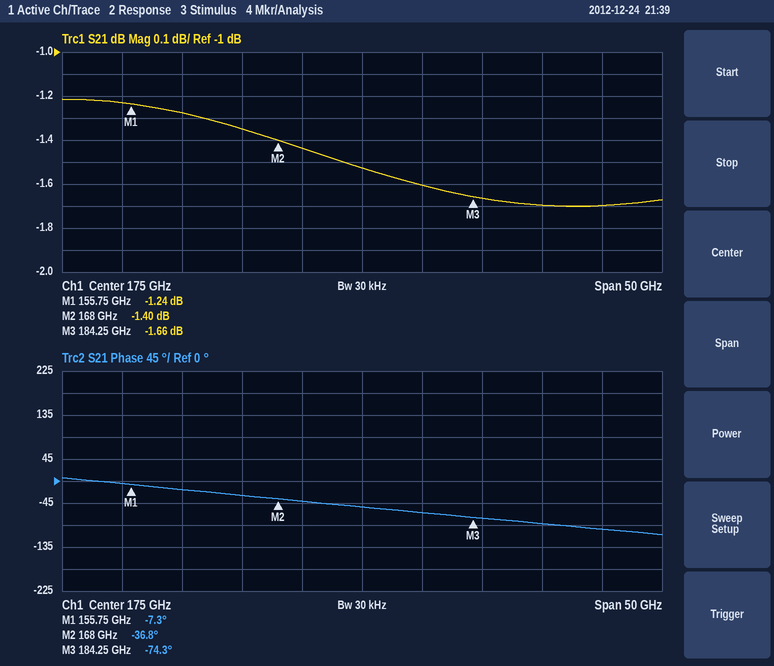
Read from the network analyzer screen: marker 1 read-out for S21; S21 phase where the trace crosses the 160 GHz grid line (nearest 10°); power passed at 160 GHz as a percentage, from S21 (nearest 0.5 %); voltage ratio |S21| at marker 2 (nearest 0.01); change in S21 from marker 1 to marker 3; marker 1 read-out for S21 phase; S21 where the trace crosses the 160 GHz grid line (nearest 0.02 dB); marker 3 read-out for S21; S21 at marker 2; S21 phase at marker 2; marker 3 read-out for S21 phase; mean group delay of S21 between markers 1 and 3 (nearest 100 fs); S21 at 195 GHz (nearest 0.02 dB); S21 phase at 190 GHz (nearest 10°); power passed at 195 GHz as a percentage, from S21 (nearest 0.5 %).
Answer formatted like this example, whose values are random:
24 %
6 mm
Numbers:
-1.24 dB
-20°
74.5 %
0.85
-0.42 dB
-7.3°
-1.28 dB
-1.66 dB
-1.40 dB
-36.8°
-74.3°
6.5 ps
-1.70 dB
-90°
67.5 %
